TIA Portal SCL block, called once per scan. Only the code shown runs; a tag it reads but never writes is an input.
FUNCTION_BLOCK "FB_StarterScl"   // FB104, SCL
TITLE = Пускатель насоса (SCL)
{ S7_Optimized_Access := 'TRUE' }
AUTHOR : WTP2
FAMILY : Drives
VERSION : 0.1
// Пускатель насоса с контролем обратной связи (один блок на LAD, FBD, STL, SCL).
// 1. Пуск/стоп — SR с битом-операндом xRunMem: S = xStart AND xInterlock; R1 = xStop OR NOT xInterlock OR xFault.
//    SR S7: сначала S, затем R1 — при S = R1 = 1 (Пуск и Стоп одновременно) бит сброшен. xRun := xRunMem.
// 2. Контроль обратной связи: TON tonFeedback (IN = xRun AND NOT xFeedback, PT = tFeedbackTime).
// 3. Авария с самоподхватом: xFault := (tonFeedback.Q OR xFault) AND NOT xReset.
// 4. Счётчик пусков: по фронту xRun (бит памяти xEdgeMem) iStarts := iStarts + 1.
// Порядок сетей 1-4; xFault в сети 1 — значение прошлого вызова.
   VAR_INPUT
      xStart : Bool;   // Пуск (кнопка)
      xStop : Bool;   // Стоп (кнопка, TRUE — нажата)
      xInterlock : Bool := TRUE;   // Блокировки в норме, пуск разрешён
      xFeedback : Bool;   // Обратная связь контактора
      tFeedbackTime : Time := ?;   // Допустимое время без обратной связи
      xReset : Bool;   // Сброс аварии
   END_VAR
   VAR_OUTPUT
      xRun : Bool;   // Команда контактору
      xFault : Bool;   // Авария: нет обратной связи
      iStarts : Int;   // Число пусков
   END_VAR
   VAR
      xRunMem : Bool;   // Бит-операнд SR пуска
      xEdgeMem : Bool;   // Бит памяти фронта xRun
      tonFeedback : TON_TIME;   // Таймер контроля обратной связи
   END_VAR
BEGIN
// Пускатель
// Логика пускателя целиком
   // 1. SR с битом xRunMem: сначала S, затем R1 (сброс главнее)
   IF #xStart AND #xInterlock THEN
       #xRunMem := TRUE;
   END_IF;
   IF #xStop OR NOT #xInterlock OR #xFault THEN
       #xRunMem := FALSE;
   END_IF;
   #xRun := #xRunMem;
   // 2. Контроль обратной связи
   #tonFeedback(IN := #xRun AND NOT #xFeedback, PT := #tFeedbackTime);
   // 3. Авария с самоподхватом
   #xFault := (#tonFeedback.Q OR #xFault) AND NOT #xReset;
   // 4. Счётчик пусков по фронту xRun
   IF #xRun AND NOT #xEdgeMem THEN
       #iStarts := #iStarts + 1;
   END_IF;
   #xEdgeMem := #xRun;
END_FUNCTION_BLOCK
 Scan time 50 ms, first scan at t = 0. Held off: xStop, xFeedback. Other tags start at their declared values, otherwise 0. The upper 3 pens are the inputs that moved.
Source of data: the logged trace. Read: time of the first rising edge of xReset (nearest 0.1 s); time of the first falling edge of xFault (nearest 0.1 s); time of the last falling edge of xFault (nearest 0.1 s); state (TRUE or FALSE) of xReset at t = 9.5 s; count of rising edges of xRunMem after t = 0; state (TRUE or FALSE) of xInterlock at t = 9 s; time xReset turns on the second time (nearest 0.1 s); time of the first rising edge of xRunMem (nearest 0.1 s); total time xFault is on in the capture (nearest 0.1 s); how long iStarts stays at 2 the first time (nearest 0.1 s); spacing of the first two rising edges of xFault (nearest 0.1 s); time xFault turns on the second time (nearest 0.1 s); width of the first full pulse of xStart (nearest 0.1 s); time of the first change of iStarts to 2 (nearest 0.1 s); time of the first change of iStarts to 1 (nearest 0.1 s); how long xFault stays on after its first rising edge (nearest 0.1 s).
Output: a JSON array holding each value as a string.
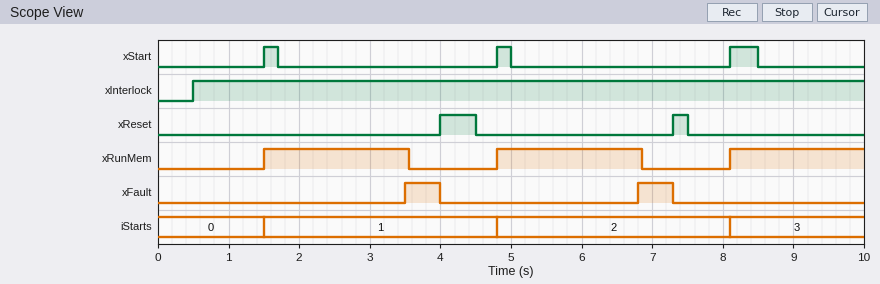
["4.0 s", "4.0 s", "7.3 s", "FALSE", "3", "TRUE", "7.3 s", "1.5 s", "1.0 s", "3.3 s", "3.3 s", "6.8 s", "0.2 s", "4.8 s", "1.5 s", "0.5 s"]
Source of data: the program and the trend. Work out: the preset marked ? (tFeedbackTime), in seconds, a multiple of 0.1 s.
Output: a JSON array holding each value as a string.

["2.0 s"]
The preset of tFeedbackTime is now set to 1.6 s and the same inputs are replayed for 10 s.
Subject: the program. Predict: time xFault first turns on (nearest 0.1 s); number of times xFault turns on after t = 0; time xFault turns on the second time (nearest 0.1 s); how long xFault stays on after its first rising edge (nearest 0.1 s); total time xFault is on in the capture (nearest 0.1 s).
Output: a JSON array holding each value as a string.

["3.1 s", "3", "6.4 s", "0.9 s", "2.1 s"]
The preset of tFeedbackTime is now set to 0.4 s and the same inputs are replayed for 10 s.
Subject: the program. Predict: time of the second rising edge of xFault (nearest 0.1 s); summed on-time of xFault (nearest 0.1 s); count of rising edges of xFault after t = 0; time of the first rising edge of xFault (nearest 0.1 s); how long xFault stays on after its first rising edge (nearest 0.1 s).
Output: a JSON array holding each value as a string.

["5.2 s", "5.7 s", "3", "1.9 s", "2.1 s"]
